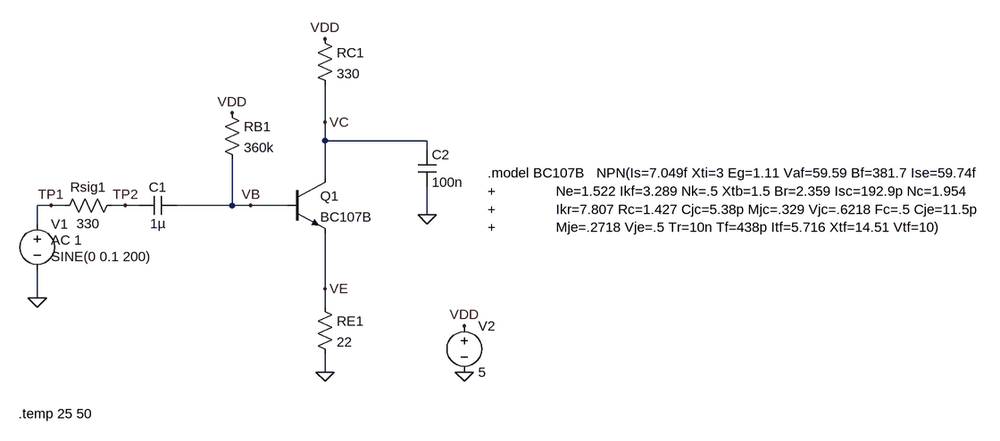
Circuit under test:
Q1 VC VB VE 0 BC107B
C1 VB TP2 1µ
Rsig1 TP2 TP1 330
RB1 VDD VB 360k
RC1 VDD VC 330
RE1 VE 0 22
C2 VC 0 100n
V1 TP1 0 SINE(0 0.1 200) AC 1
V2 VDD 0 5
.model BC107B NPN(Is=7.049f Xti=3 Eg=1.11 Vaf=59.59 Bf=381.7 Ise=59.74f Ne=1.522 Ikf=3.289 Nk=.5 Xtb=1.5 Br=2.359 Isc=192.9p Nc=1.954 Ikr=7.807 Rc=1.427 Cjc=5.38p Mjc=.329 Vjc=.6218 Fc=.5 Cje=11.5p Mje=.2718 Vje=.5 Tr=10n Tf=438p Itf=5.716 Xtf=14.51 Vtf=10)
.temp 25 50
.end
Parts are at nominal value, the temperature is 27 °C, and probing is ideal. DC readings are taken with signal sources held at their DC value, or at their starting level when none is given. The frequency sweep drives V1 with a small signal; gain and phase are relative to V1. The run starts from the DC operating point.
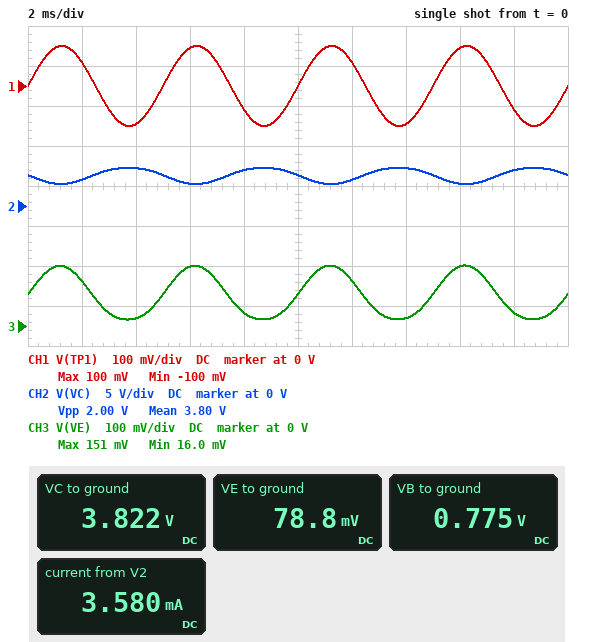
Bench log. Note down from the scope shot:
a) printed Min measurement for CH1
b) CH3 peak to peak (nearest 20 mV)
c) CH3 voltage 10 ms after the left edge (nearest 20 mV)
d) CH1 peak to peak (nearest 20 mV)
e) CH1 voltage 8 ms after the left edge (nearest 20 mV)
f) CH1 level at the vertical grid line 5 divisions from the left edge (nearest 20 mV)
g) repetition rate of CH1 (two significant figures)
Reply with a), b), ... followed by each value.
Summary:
a) -100 mV
b) 140 mV
c) 80 mV
d) 200 mV
e) -60 mV
f) 0 V
g) 200 Hz
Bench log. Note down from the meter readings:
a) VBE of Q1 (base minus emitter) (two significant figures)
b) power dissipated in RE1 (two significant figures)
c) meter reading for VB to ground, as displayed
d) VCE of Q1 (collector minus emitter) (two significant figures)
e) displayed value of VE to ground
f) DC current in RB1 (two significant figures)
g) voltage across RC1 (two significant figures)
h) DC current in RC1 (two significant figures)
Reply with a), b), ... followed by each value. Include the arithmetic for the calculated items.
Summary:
a) 775 mV - 78.8 mV = 700 mV
b) (78.8 mV)^2 / 22 Ω = 280 µW
c) 0.775 V
d) 3.822 V - 78.8 mV = 3.7 V
e) 78.8 mV
f) (5 V - 775 mV) / 360 kΩ = 12 µA
g) 5 V - 3.822 V = 1.2 V
h) (5 V - 3.822 V) / 330 Ω = 3.6 mA
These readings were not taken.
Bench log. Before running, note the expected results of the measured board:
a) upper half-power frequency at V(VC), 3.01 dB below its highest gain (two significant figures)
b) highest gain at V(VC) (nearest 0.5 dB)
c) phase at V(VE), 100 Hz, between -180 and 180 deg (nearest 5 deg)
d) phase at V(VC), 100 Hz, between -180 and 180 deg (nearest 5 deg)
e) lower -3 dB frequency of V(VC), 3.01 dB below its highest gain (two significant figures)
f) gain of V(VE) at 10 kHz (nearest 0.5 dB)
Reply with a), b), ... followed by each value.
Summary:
a) 4.9 kHz
b) 20.5 dB
c) 10 deg
d) -170 deg
e) 16 Hz
f) -3.0 dB
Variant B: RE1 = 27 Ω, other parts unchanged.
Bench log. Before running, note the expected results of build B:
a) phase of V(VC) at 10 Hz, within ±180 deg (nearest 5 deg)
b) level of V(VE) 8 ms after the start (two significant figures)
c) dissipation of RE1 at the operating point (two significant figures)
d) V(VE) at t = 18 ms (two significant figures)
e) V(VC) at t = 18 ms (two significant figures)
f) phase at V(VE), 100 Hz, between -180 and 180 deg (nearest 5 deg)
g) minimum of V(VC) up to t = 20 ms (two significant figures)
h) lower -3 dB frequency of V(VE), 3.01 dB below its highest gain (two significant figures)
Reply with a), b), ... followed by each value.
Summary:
a) -125 deg
b) 47 mV
c) 340 µW
d) 48 mV
e) 4.4 V
f) 10 deg
g) 2.9 V
h) 14 Hz
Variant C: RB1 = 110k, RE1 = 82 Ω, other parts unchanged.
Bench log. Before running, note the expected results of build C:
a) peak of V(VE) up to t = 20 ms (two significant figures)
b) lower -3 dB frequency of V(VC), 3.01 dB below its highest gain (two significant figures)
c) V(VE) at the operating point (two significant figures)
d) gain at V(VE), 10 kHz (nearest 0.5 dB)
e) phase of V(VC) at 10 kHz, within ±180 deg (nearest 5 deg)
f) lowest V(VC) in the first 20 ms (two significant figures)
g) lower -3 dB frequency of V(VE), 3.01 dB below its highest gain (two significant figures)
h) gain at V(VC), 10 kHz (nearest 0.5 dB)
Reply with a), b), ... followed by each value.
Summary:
a) 900 mV
b) 7.3 Hz
c) 810 mV
d) -0.5 dB
e) 115 deg
f) 1.4 V
g) 7.4 Hz
h) 4.5 dB
